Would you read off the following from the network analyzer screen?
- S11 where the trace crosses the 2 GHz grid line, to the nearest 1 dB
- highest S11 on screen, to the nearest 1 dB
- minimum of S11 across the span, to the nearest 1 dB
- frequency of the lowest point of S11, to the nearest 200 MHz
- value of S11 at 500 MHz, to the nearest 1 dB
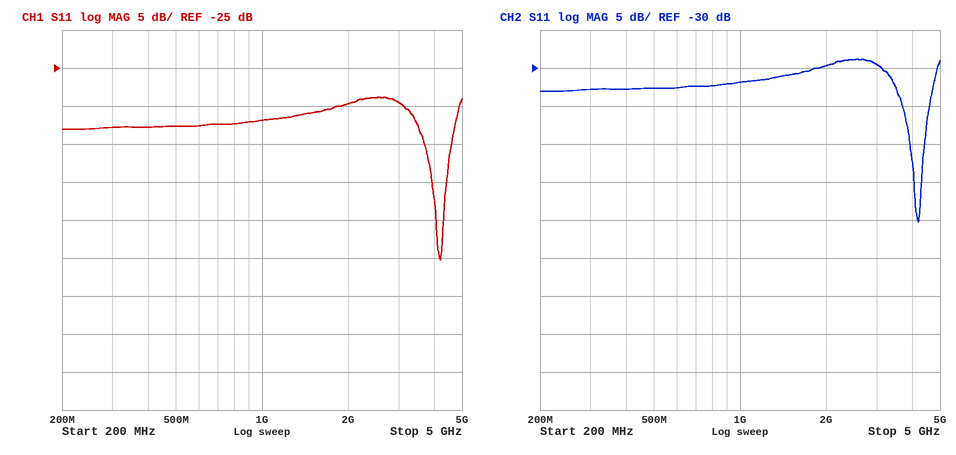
-30 dB
-29 dB
-50 dB
4.2 GHz
-33 dB
